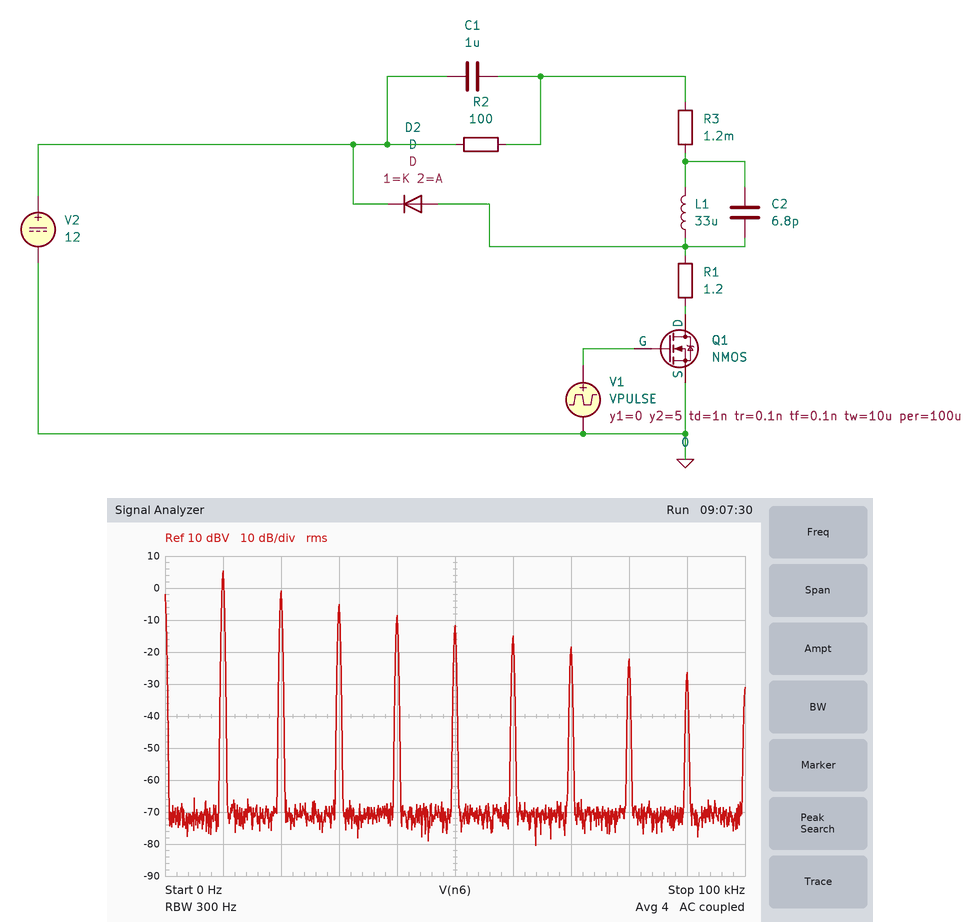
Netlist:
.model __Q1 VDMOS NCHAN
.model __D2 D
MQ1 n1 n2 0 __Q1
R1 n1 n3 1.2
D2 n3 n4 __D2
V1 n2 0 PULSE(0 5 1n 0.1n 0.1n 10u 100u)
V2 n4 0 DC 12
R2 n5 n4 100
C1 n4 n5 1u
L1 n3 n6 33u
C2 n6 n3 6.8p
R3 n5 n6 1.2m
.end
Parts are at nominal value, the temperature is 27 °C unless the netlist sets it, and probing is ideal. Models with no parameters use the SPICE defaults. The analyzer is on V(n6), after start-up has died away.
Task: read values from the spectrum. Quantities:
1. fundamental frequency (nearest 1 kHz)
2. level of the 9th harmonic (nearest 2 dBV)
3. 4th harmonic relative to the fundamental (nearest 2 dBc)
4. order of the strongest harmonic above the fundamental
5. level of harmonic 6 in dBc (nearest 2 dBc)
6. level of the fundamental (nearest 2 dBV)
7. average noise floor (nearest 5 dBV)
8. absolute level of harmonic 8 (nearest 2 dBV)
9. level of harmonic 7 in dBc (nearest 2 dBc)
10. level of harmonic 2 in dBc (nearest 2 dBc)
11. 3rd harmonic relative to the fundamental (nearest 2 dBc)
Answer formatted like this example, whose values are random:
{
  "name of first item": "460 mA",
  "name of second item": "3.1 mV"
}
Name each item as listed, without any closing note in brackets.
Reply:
{
  "fundamental frequency": "10 kHz",
  "level of the 9th harmonic": "-26 dBV",
  "4th harmonic relative to the fundamental": "-14 dBc",
  "order of the strongest harmonic above the fundamental": "2",
  "level of harmonic 6 in dBc": "-20 dBc",
  "level of the fundamental": "6 dBV",
  "average noise floor": "-70 dBV",
  "absolute level of harmonic 8": "-22 dBV",
  "level of harmonic 7 in dBc": "-24 dBc",
  "level of harmonic 2 in dBc": "-6 dBc",
  "3rd harmonic relative to the fundamental": "-10 dBc"
}
